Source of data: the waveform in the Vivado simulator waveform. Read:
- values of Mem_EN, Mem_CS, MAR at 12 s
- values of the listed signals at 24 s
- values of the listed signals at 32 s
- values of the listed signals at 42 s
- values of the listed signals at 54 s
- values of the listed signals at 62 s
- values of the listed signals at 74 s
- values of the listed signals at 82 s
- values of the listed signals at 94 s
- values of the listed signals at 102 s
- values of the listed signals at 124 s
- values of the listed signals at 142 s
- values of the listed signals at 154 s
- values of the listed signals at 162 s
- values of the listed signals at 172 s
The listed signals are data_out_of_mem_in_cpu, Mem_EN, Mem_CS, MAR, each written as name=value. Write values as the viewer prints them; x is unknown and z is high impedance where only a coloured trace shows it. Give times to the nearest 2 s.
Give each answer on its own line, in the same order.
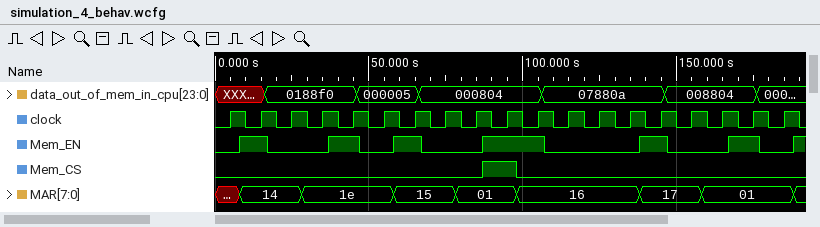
Mem_EN=1, Mem_CS=0, MAR=14
data_out_of_mem_in_cpu=0188f0, Mem_EN=0, Mem_CS=0, MAR=14
data_out_of_mem_in_cpu=0188f0, Mem_EN=0, Mem_CS=0, MAR=1e
data_out_of_mem_in_cpu=0188f0, Mem_EN=1, Mem_CS=0, MAR=1e
data_out_of_mem_in_cpu=000005, Mem_EN=0, Mem_CS=0, MAR=1e
data_out_of_mem_in_cpu=000005, Mem_EN=1, Mem_CS=0, MAR=15
data_out_of_mem_in_cpu=000804, Mem_EN=0, Mem_CS=0, MAR=15
data_out_of_mem_in_cpu=000804, Mem_EN=0, Mem_CS=0, MAR=01
data_out_of_mem_in_cpu=000804, Mem_EN=1, Mem_CS=1, MAR=01
data_out_of_mem_in_cpu=000804, Mem_EN=1, Mem_CS=0, MAR=16
data_out_of_mem_in_cpu=07880a, Mem_EN=0, Mem_CS=0, MAR=16
data_out_of_mem_in_cpu=07880a, Mem_EN=1, Mem_CS=0, MAR=17
data_out_of_mem_in_cpu=008804, Mem_EN=0, Mem_CS=0, MAR=17
data_out_of_mem_in_cpu=008804, Mem_EN=0, Mem_CS=0, MAR=01
data_out_of_mem_in_cpu=008804, Mem_EN=1, Mem_CS=0, MAR=01
